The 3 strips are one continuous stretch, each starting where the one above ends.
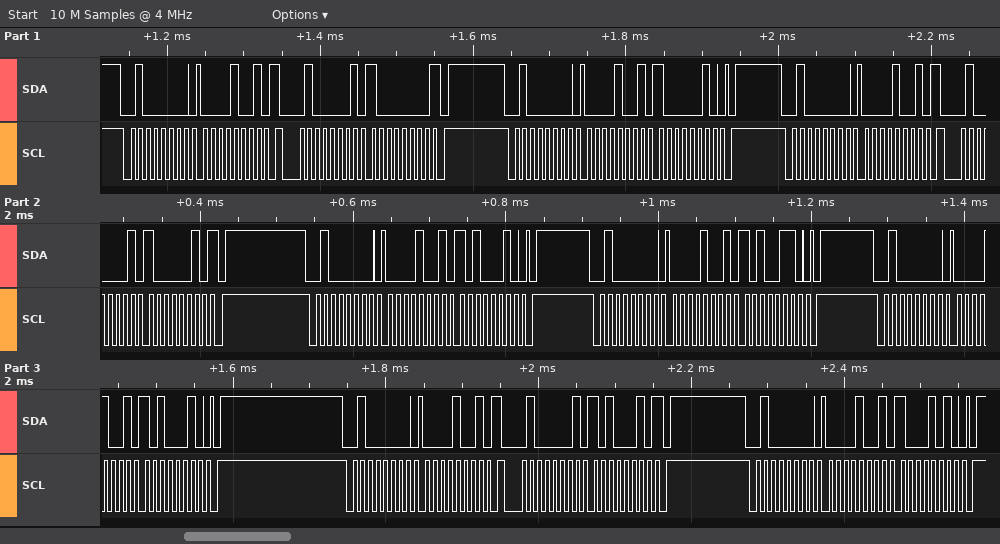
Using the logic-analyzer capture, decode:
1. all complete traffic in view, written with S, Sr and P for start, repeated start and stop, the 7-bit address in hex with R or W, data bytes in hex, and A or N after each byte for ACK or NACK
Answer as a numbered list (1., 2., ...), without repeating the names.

1. S 20W A 09 A Sr 20R A 80 N P S 20W A 09 A 82 A P S 20W A 09 A Sr 20R A 82 N P S 20W A 09 A A2 A P S 20W A 09 A A6 A P S 20W A 09 A A2 A P S 20W A 09 A Sr 20R A A2 N P S 20W A 09 A 8A A P
